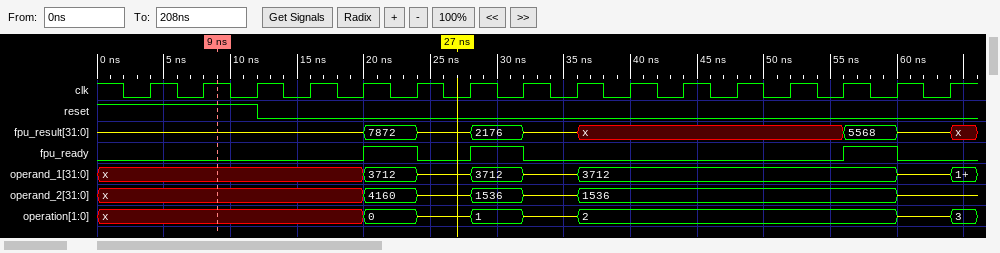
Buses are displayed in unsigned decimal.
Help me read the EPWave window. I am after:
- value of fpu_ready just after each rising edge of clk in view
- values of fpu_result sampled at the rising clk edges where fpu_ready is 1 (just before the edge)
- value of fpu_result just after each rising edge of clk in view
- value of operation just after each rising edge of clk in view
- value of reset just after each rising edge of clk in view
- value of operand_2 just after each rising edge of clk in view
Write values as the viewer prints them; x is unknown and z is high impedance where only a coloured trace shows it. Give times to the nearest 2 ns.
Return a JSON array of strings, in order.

["0 0 0 0 1 0 1 0 0 0 0 0 0 1 0 0", "7872, 2176, 5568", "z, z, z, z, 7872, z, 2176, z, x, x, x, x, x, 5568, z, x", "x, x, x, x, 0, z, 1, z, 2, 2, 2, 2, 2, 2, z, 3", "1 1 0 0 0 0 0 0 0 0 0 0 0 0 0 0", "x, x, x, x, 4160, z, 1536, z, 1536, 1536, 1536, 1536, 1536, 1536, z, z"]
